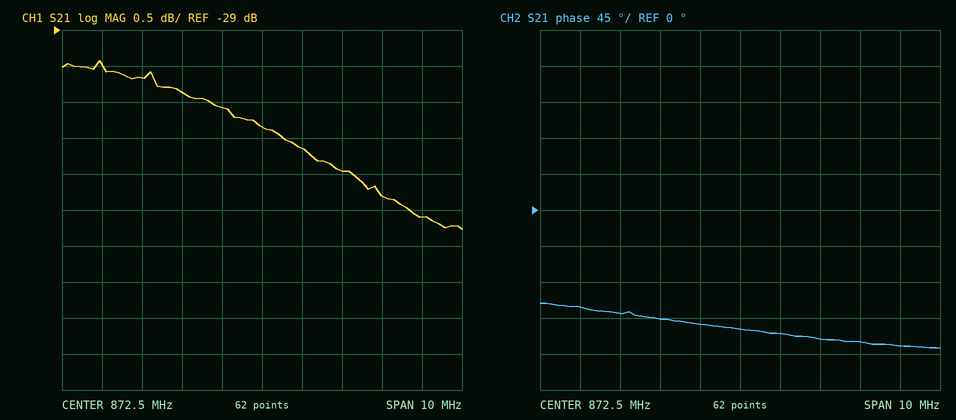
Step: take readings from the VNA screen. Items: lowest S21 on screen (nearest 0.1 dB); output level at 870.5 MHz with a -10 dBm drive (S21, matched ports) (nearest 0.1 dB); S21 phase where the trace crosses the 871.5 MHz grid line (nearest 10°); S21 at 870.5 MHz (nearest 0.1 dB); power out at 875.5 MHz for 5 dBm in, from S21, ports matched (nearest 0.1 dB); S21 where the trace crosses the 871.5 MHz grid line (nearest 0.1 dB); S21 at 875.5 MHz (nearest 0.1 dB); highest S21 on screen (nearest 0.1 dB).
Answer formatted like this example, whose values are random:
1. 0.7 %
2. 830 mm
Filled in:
1. -31.8 dB
2. -39.9 dBm
3. -140°
4. -29.9 dB
5. -26.3 dBm
6. -30.1 dB
7. -31.3 dB
8. -29.4 dB
